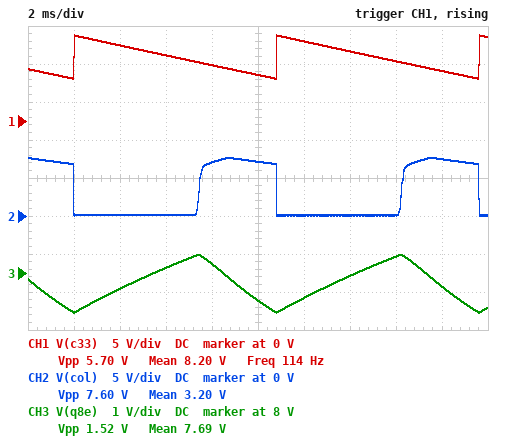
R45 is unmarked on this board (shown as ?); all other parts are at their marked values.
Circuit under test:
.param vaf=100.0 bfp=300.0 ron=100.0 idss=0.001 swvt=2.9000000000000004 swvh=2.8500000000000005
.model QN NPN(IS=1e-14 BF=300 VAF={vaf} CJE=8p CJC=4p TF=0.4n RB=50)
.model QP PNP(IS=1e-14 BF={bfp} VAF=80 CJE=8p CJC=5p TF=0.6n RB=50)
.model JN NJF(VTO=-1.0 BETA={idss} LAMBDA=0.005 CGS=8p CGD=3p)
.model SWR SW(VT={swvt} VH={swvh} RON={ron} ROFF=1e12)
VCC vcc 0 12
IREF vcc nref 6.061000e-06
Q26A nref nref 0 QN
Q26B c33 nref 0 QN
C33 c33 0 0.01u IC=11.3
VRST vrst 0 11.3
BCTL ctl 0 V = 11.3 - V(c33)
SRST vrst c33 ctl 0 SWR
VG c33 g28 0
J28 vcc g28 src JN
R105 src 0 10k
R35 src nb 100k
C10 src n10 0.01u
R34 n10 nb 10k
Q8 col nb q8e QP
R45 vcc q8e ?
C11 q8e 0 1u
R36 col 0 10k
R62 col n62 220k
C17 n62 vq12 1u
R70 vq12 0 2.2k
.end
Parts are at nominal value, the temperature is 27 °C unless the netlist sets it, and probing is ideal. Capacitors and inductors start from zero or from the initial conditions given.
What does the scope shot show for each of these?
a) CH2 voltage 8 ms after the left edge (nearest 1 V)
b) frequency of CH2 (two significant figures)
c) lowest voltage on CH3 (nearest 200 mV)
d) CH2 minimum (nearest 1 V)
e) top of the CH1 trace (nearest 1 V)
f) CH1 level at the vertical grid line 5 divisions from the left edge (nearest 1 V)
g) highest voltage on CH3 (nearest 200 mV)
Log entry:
7 V
110 Hz
7.0 V
0 V
11 V
6 V
8.4 V
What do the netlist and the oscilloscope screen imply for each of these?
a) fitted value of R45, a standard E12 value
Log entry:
15 kΩ
